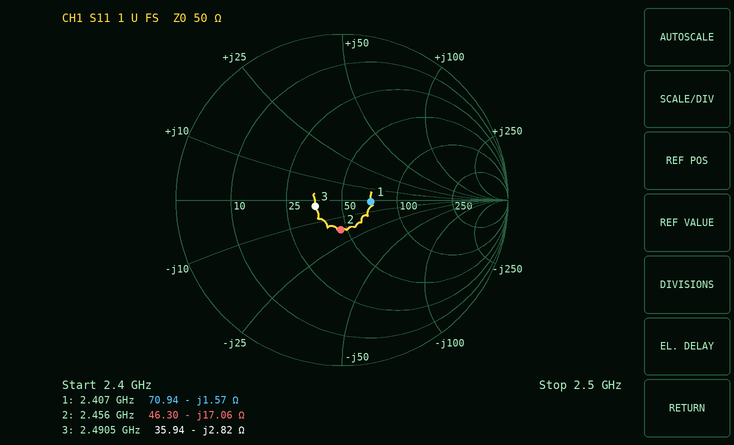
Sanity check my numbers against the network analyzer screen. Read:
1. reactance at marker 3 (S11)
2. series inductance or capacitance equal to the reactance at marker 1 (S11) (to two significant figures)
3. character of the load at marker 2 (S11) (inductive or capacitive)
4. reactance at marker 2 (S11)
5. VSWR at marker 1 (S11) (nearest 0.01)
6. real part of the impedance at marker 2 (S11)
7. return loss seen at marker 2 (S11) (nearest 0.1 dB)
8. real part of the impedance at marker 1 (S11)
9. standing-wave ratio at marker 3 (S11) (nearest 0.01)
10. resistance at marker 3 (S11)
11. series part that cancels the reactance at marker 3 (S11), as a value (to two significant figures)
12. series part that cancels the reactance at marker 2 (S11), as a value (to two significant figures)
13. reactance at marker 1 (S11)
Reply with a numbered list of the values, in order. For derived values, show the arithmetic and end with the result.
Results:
1. -2.82 Ω
2. C = 1/(2π × 2.407 GHz × 1.57 Ω) ≈ 42 pF
3. capacitive
4. -17.06 Ω
5. 1.42
6. 46.30 Ω
7. 15.0 dB
8. 70.94 Ω
9. 1.40
10. 35.94 Ω
11. L = 2.82 Ω/(2π × 2.4905 GHz) ≈ 180 pH
12. L = 17.06 Ω/(2π × 2.456 GHz) ≈ 1.1 nH
13. -1.57 Ω
